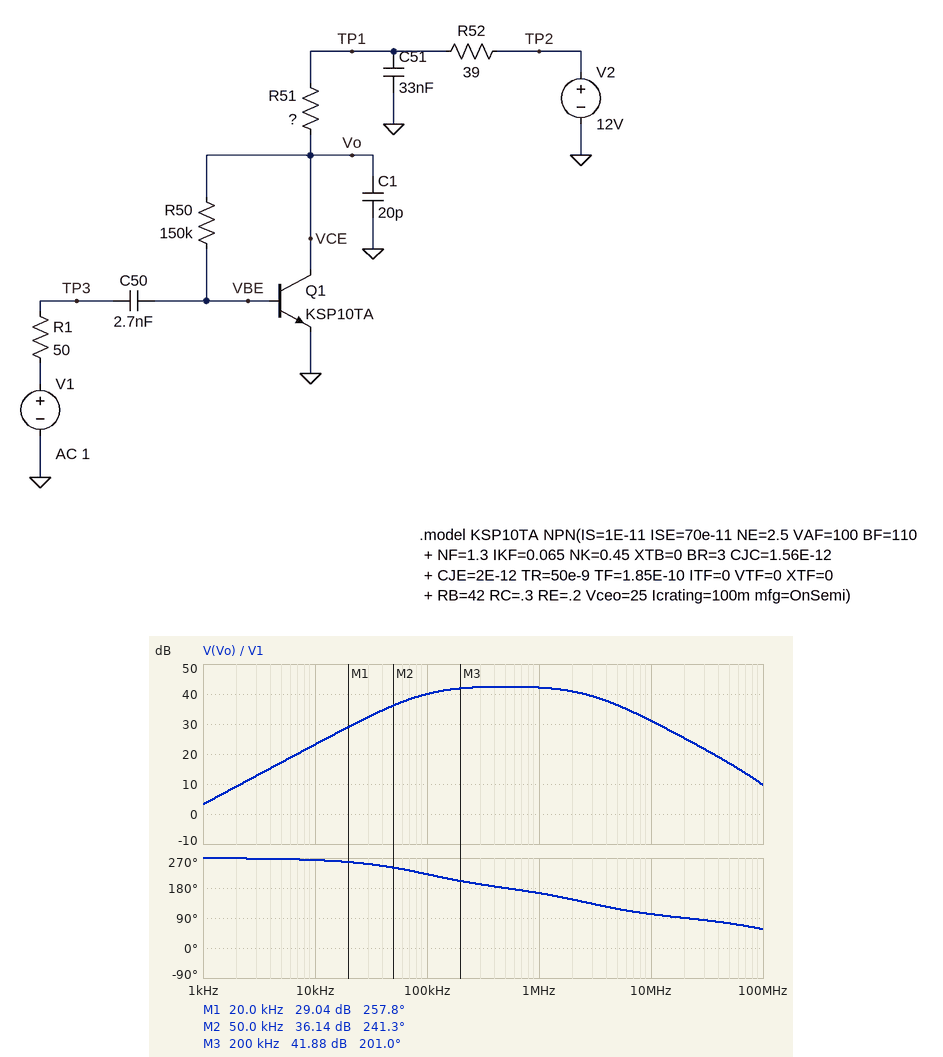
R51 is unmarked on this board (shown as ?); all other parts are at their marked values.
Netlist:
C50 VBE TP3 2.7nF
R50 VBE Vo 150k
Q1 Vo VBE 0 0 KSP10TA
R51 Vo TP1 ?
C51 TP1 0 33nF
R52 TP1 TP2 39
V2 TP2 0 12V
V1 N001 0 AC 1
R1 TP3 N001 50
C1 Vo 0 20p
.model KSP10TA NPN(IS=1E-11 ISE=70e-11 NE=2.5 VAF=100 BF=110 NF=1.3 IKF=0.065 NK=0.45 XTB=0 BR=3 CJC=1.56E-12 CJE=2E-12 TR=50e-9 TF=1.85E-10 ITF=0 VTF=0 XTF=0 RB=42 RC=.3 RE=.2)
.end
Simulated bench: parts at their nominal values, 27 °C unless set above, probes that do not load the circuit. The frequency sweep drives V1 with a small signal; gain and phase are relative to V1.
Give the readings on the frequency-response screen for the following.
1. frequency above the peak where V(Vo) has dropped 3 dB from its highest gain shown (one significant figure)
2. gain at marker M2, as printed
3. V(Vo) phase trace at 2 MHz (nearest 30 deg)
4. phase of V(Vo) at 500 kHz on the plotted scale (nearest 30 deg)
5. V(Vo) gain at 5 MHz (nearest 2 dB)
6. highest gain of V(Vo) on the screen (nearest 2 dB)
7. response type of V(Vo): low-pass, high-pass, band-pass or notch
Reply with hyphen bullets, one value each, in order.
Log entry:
- 3 MHz
- 36.14 dB
- 150 deg
- 180 deg
- 36 dB
- 42 dB
- band-pass
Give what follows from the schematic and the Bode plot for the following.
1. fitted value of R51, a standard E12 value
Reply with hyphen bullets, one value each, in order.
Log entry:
- 2.7 kΩ
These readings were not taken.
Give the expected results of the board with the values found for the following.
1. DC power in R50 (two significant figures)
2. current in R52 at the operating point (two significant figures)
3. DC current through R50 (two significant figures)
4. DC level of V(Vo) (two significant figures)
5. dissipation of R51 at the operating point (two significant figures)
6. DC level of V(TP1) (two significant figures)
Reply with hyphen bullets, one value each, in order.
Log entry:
- 180 µW
- 2.2 mA
- 35 µA
- 5.9 V
- 14 mW
- 12 V
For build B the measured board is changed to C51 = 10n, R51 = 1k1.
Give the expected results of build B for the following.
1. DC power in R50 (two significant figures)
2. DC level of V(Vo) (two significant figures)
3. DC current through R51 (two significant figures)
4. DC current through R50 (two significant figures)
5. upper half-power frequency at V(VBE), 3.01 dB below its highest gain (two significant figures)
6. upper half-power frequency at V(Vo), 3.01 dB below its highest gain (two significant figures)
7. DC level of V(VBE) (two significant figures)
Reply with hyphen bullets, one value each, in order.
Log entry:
- 360 µW
- 8.0 V
- 3.5 mA
- 49 µA
- 140 MHz
- 6.0 MHz
- 660 mV
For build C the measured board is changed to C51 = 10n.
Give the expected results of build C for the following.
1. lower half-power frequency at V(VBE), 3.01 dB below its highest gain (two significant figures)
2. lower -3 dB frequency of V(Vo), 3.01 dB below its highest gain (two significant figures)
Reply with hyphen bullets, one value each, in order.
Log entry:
- 95 kHz
- 89 kHz
